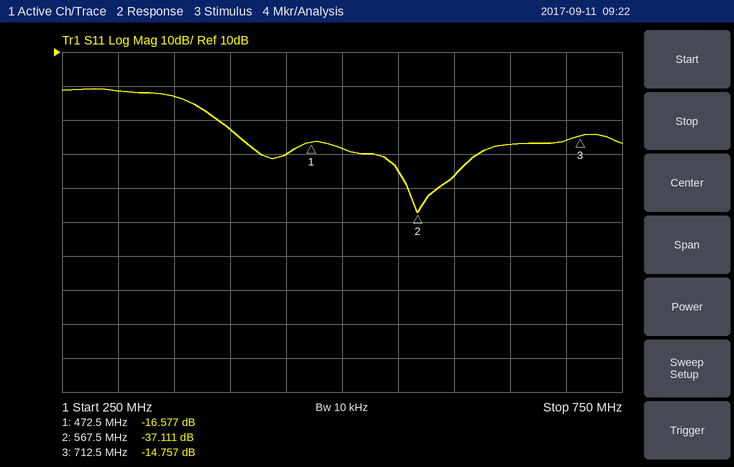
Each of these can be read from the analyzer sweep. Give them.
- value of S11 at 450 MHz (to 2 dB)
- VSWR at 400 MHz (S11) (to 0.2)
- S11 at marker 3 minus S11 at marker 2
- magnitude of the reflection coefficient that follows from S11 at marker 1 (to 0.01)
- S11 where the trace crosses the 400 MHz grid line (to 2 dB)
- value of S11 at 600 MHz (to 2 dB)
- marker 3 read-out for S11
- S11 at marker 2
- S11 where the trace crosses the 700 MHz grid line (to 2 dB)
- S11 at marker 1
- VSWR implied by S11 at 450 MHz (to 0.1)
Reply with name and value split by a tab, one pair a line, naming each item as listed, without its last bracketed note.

value of S11 at 450 MHz	-20 dB
VSWR at 400 MHz (S11)	1.6
S11 at marker 3 minus S11 at marker 2	22.354 dB
magnitude of the reflection coefficient that follows from S11 at marker 1	0.15
S11 where the trace crosses the 400 MHz grid line	-12 dB
value of S11 at 600 MHz	-26 dB
marker 3 read-out for S11	-14.757 dB
S11 at marker 2	-37.111 dB
S11 where the trace crosses the 700 MHz grid line	-16 dB
S11 at marker 1	-16.577 dB
VSWR implied by S11 at 450 MHz	1.2
